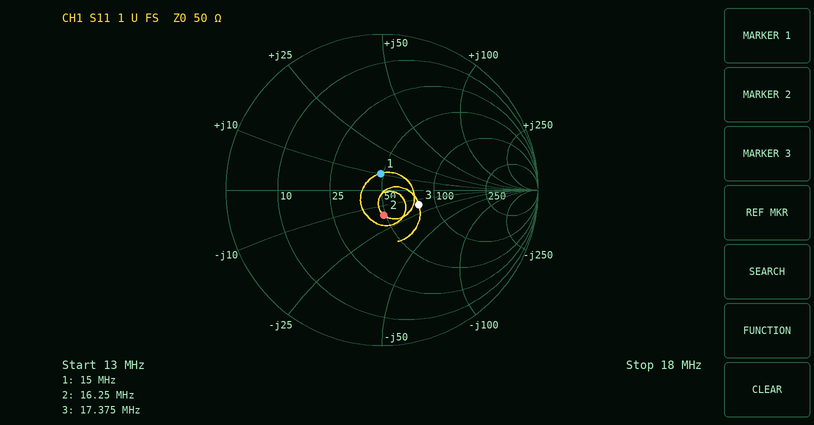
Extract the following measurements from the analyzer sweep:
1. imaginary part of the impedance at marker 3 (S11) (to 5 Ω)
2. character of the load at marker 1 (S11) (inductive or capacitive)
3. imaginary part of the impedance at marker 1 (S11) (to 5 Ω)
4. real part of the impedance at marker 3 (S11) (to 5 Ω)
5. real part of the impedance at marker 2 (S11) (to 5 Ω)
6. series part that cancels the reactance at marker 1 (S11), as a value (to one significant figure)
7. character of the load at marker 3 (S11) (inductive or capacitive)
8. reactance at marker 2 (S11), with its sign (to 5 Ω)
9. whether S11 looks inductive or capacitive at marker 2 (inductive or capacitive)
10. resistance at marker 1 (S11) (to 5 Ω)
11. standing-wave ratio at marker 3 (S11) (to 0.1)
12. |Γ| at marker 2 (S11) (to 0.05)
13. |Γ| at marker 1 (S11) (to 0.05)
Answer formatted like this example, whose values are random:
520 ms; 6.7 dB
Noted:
-15 Ω; inductive; +10 Ω; 80 Ω; 50 Ω; 1 nF; capacitive; -15 Ω; capacitive; 50 Ω; 1.7; 0.15; 0.10
